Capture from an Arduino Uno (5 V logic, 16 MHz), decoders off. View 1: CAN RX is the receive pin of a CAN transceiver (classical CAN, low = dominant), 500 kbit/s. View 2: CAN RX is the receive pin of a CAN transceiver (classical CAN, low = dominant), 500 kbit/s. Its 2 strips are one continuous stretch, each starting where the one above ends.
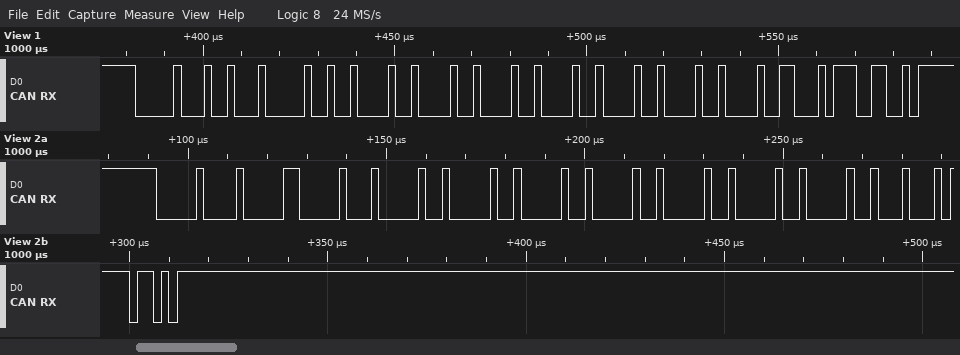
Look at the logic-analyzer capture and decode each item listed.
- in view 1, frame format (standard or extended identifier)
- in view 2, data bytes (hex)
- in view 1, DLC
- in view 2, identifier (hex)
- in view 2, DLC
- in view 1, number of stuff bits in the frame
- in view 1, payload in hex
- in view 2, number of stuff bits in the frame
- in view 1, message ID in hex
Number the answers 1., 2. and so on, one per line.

1. standard
2. 04 04 04 04 04 04 04 04
3. 8
4. 0x004
5. 8
6. 2
7. 09 09 09 09 09 09 09 09
8. 10
9. 0x009
